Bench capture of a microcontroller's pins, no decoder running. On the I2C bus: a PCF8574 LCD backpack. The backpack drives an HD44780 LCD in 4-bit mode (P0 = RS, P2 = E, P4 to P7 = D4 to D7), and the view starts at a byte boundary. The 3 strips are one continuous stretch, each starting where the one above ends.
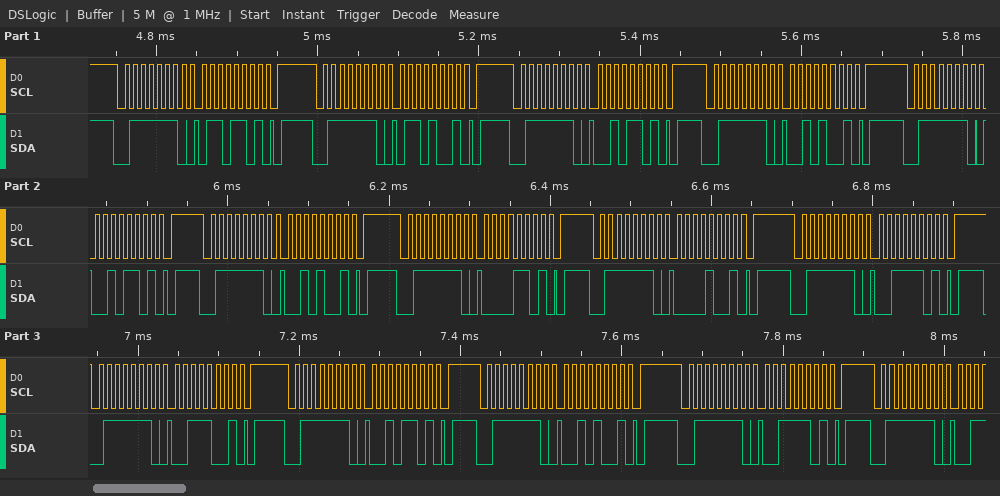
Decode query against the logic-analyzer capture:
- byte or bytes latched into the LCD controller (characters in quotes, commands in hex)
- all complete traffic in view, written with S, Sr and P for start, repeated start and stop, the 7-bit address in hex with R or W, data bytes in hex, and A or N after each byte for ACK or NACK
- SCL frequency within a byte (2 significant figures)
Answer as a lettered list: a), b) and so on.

a) 'b' ' ' '2'
b) S 3FW A 6D A P S 3FW A 69 A P S 3FW A 2D A P S 3FW A 29 A P S 3FW A 2D A P S 3FW A 29 A P S 3FW A 0D A P S 3FW A 09 A P S 3FW A 3D A P S 3FW A 39 A P S 3FW A 2D A P S 3FW A 29 A P S 3FW A 3D A P S 3FW A
c) 100 kHz
